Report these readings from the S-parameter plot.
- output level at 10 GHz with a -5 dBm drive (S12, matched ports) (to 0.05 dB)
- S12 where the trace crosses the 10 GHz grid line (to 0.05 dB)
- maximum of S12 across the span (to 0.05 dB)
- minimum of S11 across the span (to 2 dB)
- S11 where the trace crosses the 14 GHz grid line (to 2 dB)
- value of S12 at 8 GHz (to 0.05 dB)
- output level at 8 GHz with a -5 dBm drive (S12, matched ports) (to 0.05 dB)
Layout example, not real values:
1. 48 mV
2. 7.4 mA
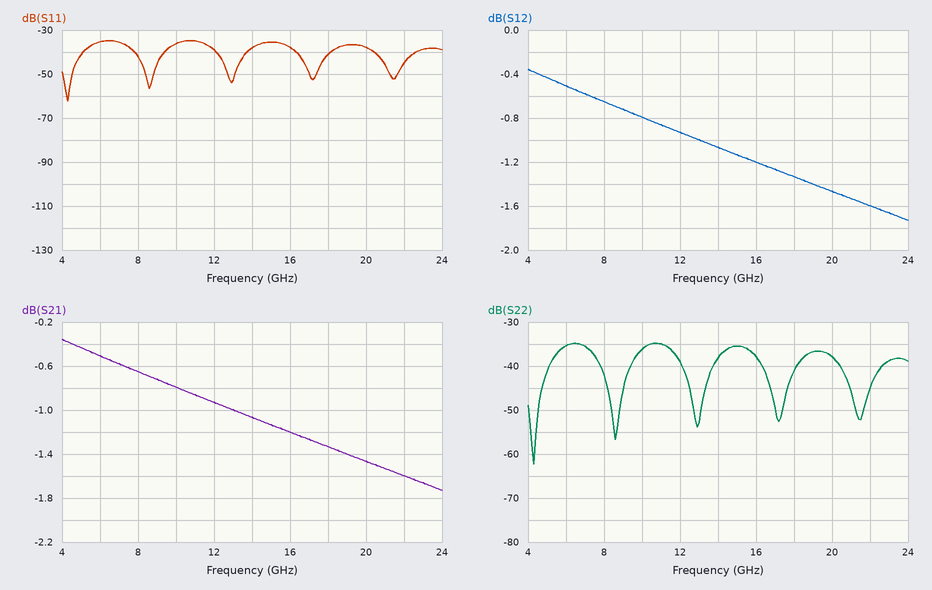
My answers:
1. -5.80 dBm
2. -0.80 dB
3. -0.35 dB
4. -62 dB
5. -38 dB
6. -0.65 dB
7. -5.65 dBm
